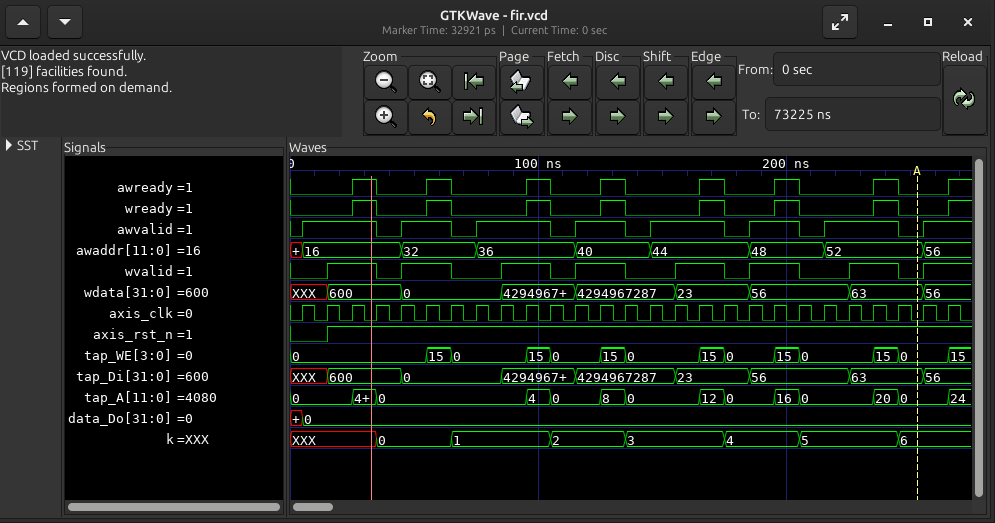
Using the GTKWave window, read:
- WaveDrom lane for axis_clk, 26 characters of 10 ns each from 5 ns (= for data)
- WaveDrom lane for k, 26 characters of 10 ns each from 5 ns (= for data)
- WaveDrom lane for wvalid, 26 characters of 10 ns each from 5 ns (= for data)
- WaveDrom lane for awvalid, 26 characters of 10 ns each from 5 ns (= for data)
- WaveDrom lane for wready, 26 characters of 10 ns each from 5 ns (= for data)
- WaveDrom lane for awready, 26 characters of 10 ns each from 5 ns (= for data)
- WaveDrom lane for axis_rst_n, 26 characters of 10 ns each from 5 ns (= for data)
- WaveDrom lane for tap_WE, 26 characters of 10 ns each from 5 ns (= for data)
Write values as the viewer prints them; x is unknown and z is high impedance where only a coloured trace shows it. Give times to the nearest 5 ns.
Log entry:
{name: 'axis_clk', wave: 'p.........................'}
{name: 'k', wave: 'x..=..=...=..=...=..=...=.', data: '0 1 2 3 4 5 6'}
{name: 'wvalid', wave: '01.01.0.1.01.0.1.01.0.1.01'}
{name: 'awvalid', wave: '1..01.01..01.01..01.01..01'}
{name: 'wready', wave: '0.10.10..10.10..10.10..10.'}
{name: 'awready', wave: '0.10.10..10.10..10.10..10.'}
{name: 'axis_rst_n', wave: '01........................'}
{name: 'tap_WE', wave: '=....==..==.==..==.==..==.', data: '0 15 0 15 0 15 0 15 0 15 0 15 0'}
